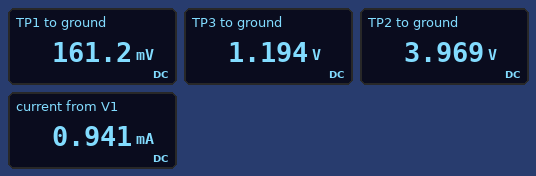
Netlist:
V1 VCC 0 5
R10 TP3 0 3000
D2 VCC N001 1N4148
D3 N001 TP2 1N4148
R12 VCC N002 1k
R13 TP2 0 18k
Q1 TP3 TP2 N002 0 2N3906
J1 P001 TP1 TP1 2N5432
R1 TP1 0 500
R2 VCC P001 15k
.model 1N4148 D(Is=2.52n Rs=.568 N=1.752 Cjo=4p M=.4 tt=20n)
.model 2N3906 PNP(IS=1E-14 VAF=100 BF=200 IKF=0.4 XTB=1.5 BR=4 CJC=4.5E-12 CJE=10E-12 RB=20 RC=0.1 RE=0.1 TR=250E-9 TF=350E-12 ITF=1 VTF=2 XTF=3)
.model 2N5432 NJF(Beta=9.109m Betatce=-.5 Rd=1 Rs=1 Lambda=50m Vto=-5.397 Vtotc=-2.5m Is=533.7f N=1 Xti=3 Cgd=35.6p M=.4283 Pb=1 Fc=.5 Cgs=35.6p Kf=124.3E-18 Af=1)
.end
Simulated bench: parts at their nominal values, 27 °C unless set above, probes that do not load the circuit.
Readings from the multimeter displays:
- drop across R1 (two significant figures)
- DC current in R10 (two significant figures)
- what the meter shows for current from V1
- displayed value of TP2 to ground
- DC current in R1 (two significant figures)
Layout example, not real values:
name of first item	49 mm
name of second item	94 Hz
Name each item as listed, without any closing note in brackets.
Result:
drop across R1	160 mV
DC current in R10	400 µA
what the meter shows for current from V1	0.941 mA
displayed value of TP2 to ground	3.969 V
DC current in R1	320 µA
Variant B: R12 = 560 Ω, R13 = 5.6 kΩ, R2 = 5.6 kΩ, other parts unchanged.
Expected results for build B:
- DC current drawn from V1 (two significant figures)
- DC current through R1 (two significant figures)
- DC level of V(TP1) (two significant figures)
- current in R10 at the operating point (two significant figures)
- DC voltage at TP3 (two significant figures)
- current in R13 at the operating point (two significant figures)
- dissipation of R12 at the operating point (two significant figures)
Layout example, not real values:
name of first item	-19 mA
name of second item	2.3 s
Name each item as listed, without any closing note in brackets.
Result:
DC current drawn from V1	2.4 mA
DC current through R1	820 µA
DC level of V(TP1)	410 mV
current in R10 at the operating point	860 µA
DC voltage at TP3	2.6 V
current in R13 at the operating point	690 µA
dissipation of R12 at the operating point	420 µW
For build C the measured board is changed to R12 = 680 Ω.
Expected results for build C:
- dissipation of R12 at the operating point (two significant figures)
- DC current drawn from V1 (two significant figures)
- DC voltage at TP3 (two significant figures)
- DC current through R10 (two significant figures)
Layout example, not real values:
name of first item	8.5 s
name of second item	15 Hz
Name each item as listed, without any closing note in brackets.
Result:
dissipation of R12 at the operating point	220 µW
DC current drawn from V1	1.1 mA
DC voltage at TP3	1.7 V
DC current through R10	570 µA
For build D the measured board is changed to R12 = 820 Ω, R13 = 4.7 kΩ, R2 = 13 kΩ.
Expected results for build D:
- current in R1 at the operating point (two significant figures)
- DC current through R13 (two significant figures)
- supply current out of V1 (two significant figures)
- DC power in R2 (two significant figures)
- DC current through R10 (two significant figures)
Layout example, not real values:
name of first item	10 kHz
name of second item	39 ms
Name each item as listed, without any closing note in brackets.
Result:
current in R1 at the operating point	370 µA
DC current through R13	820 µA
supply current out of V1	1.8 mA
DC power in R2	1.8 mW
DC current through R10	620 µA
